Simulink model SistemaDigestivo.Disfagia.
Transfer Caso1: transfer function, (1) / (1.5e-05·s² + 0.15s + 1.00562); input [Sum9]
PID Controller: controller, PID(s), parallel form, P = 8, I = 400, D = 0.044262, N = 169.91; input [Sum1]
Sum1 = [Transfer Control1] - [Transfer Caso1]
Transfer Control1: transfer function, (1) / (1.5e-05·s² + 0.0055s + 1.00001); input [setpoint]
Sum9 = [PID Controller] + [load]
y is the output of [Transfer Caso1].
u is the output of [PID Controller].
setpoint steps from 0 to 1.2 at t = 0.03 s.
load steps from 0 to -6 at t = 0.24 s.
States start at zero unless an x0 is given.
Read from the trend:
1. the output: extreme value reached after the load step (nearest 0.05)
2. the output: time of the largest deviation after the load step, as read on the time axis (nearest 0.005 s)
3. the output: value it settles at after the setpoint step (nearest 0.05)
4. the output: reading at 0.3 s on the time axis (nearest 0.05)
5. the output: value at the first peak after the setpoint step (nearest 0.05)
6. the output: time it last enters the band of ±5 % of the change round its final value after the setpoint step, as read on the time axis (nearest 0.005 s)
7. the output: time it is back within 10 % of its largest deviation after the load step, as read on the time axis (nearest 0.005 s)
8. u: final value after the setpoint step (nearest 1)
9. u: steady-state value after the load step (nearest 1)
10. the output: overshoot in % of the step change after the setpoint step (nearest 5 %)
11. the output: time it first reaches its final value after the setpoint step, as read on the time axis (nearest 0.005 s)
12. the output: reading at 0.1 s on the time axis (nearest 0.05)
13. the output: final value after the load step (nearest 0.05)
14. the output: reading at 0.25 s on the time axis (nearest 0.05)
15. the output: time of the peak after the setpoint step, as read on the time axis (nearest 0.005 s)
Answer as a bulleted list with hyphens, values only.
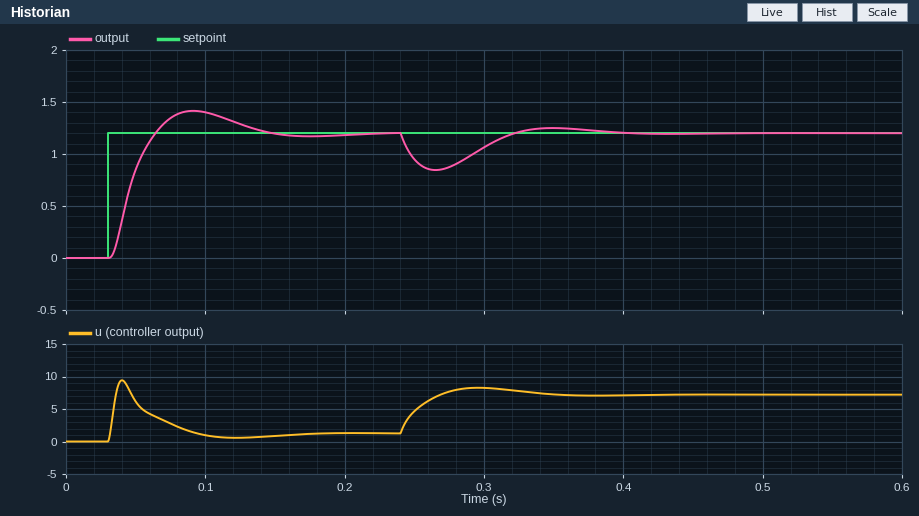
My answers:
- 0.85
- 0.265 s
- 1.20
- 1.05
- 1.40
- 0.130 s
- 0.370 s
- 1
- 7
- 20 %
- 0.065 s
- 1.40
- 1.20
- 0.95
- 0.090 s
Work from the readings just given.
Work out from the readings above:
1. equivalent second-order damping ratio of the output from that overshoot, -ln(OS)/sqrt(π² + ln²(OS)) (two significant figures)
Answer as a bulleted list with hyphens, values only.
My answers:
- 0.46
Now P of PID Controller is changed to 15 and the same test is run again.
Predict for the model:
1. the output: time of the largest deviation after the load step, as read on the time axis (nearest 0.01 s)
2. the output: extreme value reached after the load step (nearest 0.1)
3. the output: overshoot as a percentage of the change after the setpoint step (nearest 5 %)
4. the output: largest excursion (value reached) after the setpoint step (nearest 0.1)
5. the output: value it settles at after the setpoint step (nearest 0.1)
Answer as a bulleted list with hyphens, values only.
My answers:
- 0.26 s
- 0.9
- 10 %
- 1.3
- 1.2
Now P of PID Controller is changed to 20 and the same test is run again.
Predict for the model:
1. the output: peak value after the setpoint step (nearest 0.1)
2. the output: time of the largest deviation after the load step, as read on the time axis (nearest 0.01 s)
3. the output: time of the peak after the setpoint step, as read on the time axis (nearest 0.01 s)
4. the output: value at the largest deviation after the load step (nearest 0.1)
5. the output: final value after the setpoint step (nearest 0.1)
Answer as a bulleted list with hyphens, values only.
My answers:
- 1.3
- 0.26 s
- 0.08 s
- 1.0
- 1.2
